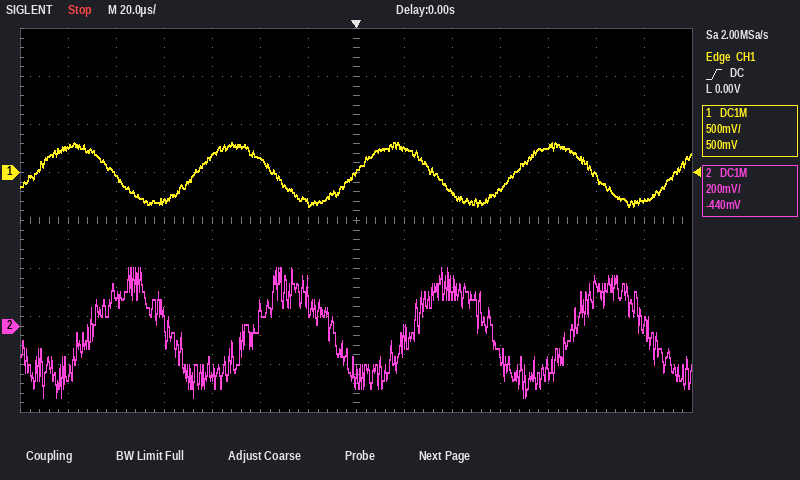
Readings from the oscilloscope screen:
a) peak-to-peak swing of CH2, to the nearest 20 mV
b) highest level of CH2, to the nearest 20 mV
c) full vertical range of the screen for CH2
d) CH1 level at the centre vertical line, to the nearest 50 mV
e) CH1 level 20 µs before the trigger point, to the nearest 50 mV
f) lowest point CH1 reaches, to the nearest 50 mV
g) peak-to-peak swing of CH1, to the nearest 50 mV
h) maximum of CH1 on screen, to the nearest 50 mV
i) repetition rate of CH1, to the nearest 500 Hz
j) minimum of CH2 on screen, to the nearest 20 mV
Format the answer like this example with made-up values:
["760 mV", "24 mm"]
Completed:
["540 mV", "240 mV", "1.6 V", "0 mV", "-300 mV", "-350 mV", "650 mV", "300 mV", "15.0 kHz", "-300 mV"]
